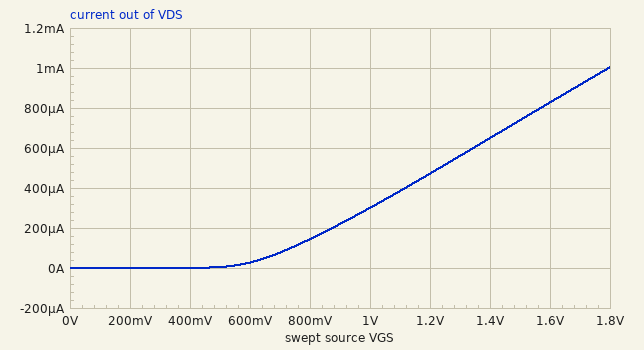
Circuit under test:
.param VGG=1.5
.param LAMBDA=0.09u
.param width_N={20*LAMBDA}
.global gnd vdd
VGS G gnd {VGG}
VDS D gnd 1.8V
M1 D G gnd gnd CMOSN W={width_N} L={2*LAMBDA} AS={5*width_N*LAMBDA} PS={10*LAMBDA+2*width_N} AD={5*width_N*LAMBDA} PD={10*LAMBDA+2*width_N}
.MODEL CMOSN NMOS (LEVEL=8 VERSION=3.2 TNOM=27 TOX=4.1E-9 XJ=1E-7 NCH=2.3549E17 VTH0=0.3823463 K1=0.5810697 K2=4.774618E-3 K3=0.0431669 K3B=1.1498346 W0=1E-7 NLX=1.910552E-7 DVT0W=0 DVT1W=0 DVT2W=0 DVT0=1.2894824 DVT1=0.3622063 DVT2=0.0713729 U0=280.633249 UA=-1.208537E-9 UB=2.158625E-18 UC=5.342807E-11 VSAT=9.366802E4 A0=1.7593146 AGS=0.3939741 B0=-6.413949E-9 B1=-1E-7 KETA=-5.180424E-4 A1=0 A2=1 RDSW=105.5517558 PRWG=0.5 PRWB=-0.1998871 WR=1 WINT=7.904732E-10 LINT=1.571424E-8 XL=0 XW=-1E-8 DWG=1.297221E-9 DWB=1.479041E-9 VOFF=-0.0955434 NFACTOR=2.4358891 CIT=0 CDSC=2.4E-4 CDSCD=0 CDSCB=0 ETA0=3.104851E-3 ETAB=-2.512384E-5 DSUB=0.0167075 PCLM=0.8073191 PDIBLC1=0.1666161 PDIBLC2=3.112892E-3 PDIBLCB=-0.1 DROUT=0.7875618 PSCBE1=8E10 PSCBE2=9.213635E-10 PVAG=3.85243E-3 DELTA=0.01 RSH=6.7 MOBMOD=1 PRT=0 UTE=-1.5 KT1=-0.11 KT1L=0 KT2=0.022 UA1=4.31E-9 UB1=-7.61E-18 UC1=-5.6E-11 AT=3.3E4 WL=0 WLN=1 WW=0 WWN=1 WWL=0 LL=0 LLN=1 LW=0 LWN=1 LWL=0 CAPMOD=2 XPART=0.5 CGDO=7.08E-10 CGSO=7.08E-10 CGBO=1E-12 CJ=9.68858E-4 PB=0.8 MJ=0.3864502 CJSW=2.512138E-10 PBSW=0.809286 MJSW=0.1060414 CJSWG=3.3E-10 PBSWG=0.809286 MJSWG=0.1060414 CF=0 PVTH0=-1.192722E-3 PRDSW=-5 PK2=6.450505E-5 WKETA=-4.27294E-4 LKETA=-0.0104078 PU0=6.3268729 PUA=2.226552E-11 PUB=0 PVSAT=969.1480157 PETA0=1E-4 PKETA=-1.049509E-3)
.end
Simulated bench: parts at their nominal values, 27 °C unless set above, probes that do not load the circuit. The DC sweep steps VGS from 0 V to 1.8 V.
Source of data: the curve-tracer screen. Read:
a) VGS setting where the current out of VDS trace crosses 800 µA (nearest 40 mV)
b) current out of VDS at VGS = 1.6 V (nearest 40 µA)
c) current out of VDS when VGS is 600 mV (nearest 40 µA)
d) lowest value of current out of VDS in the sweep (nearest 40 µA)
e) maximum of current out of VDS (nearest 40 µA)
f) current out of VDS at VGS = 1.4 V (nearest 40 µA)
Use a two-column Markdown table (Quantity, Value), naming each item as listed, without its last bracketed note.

| Quantity | Value |
|---|---|
| VGS setting where the current out of VDS trace crosses 800 µA | 1.56 V |
| current out of VDS at VGS = 1.6 V | 840 µA |
| current out of VDS when VGS is 600 mV | 40 µA |
| lowest value of current out of VDS in the sweep | 0 A |
| maximum of current out of VDS | 1.00 mA |
| current out of VDS at VGS = 1.4 V | 640 µA |
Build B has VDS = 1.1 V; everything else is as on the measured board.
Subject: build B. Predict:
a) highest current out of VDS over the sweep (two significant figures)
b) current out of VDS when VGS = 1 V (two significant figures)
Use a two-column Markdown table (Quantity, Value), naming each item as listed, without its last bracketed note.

| Quantity | Value |
|---|---|
| highest current out of VDS over the sweep | 960 µA |
| current out of VDS when VGS = 1 V | 280 µA |
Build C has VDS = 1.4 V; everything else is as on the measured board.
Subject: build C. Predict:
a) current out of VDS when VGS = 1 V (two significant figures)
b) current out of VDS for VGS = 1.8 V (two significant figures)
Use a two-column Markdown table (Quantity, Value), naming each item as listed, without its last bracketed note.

| Quantity | Value |
|---|---|
| current out of VDS when VGS = 1 V | 290 µA |
| current out of VDS for VGS = 1.8 V | 980 µA |
